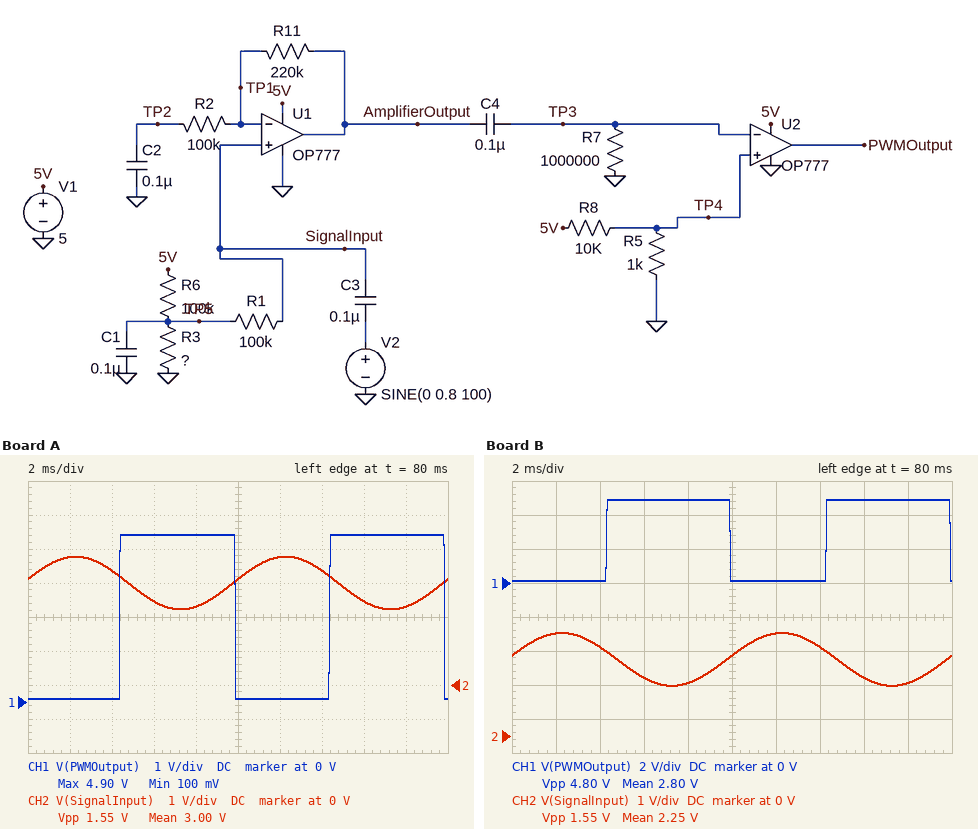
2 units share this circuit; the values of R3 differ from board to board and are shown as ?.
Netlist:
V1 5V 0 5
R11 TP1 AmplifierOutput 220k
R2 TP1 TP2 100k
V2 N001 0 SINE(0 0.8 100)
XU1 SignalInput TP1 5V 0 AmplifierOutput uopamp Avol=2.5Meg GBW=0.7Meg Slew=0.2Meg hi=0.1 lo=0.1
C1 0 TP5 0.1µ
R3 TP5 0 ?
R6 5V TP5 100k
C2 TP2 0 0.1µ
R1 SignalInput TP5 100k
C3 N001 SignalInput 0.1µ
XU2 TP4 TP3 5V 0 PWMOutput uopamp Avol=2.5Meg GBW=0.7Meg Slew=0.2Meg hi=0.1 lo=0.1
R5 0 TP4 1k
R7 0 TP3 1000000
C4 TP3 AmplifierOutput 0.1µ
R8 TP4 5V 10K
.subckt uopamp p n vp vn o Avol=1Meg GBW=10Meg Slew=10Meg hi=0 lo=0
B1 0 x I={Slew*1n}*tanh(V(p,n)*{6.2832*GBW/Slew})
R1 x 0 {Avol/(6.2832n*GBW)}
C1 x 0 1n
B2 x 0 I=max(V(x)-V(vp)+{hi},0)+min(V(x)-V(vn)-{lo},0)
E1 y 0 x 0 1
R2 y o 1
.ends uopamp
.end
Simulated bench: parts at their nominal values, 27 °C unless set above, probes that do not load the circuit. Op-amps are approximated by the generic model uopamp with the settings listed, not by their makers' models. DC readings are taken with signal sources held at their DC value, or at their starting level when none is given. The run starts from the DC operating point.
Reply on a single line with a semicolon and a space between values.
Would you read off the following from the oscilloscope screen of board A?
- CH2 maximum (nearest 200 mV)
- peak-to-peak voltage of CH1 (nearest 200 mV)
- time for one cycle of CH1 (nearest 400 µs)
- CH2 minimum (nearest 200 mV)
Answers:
3.8 V; 4.8 V; 10.0 ms; 2.2 V
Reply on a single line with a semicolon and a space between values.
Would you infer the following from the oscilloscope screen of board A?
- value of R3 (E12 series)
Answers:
150 kΩ
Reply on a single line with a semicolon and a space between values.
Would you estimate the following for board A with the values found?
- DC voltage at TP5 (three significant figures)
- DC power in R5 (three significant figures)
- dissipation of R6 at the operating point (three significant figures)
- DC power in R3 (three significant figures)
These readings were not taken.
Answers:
3.00 V; 207 µW; 40.0 µW; 60.0 µW
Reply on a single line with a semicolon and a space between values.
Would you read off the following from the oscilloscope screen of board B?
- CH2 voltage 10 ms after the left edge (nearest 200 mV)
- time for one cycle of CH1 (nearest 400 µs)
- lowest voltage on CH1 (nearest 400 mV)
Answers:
2.4 V; 10.0 ms; 0 V
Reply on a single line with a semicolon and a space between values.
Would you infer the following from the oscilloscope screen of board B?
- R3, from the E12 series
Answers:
82 kΩ
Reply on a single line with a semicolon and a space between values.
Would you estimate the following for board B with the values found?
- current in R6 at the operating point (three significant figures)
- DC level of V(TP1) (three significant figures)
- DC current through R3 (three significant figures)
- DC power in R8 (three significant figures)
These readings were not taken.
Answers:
27.5 µA; 2.25 V; 27.5 µA; 2.07 mW
